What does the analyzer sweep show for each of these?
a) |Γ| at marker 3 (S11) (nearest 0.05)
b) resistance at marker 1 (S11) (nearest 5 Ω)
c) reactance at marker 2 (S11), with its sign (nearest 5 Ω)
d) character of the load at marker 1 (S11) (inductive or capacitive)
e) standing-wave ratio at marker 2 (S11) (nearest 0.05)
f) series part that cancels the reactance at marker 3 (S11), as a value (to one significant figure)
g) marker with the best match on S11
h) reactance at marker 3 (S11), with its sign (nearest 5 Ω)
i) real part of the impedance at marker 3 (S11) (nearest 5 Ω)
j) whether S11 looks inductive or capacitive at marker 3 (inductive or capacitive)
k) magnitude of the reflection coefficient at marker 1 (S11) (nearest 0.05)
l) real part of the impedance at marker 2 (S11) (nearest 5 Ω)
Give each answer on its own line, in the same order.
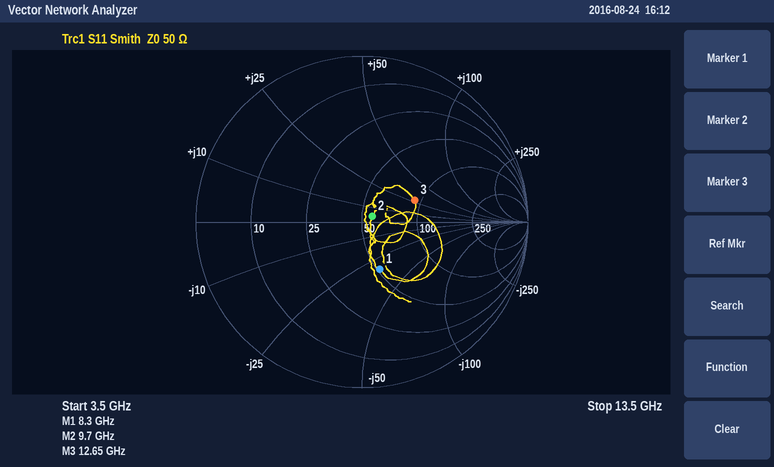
0.35
50 Ω
+5 Ω
capacitive
1.15
500 fF
marker 2
+25 Ω
90 Ω
inductive
0.30
55 Ω
